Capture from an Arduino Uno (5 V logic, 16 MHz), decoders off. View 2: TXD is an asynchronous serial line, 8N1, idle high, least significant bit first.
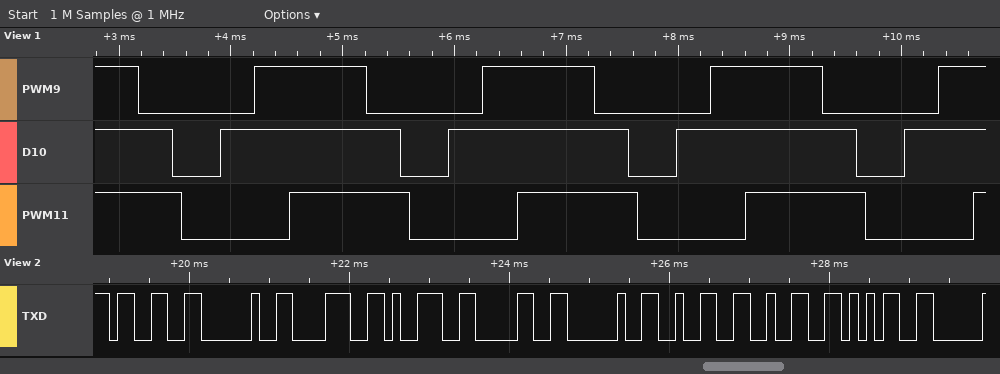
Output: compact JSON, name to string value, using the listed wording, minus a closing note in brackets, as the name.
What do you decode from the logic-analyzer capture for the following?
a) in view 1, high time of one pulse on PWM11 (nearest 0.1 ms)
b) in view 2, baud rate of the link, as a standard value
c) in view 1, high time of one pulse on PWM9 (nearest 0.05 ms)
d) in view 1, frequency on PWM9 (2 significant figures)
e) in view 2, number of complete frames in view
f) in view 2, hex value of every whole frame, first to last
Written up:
{"in view 1, high time of one pulse on PWM11": "1.1 ms", "in view 2, baud rate of the link, as a standard value": "9600 baud", "in view 1, high time of one pulse on PWM9": "1.00 ms", "in view 1, frequency on PWM9": "490 Hz", "in view 2, number of complete frames in view": "9", "in view 2, hex value of every whole frame, first to last": "33 20 38 39 30 20 32 32 35"}
